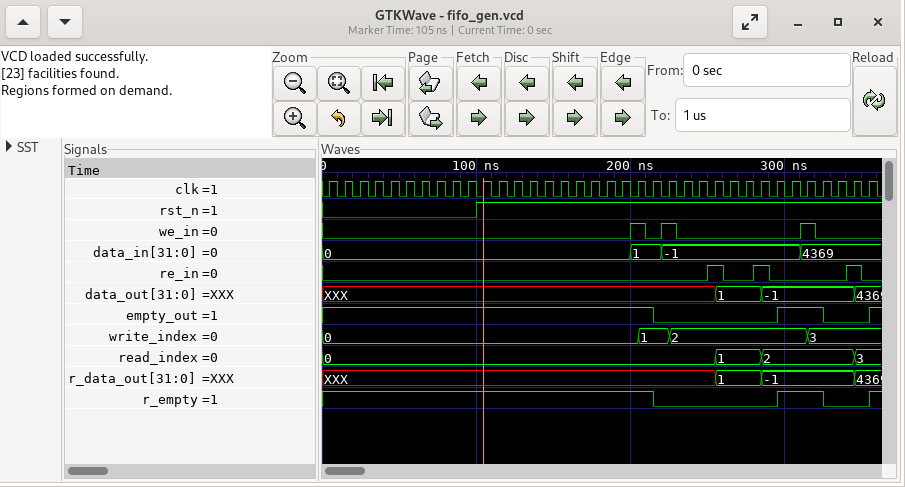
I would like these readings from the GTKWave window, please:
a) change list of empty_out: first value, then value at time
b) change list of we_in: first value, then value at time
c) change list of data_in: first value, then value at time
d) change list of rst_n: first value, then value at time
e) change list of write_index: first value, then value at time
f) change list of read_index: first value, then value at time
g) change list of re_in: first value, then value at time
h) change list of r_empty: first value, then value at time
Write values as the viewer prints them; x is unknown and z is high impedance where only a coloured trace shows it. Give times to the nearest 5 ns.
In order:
1, 0 at 215 ns, 1 at 295 ns, 0 at 325 ns, 1 at 355 ns
0, 1 at 200 ns, 0 at 210 ns, 1 at 220 ns, 0 at 230 ns, 1 at 310 ns, 0 at 320 ns
0, 1 at 200 ns, -1 at 220 ns, 4369 at 310 ns
0, 1 at 100 ns
0, 1 at 205 ns, 2 at 225 ns, 3 at 315 ns
0, 1 at 255 ns, 2 at 285 ns, 3 at 345 ns
0, 1 at 250 ns, 0 at 260 ns, 1 at 280 ns, 0 at 290 ns, 1 at 340 ns, 0 at 350 ns
1, 0 at 215 ns, 1 at 295 ns, 0 at 325 ns, 1 at 355 ns
